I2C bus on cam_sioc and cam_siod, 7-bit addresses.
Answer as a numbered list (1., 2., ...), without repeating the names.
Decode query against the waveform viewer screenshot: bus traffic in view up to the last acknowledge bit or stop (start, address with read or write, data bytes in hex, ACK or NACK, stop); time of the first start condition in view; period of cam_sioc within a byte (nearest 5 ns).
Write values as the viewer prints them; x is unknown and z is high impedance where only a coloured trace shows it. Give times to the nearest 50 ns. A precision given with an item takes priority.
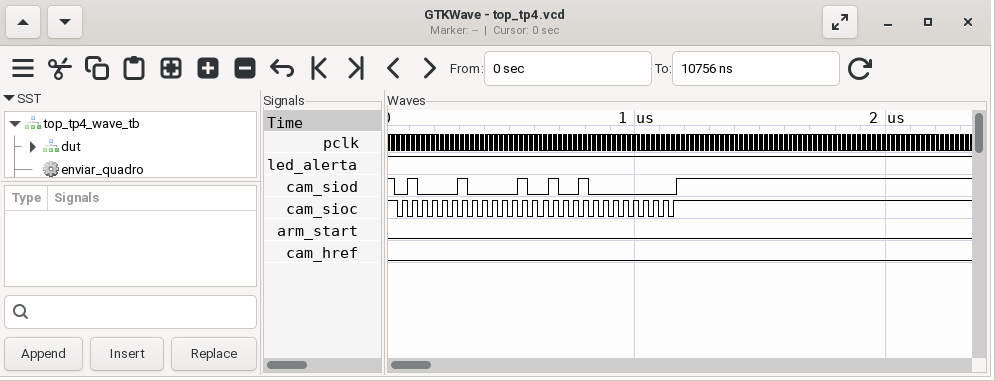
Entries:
1. start, address 21 write ACK, 12 ACK, 80 ACK, stop
2. 50 ns
3. 40 ns
